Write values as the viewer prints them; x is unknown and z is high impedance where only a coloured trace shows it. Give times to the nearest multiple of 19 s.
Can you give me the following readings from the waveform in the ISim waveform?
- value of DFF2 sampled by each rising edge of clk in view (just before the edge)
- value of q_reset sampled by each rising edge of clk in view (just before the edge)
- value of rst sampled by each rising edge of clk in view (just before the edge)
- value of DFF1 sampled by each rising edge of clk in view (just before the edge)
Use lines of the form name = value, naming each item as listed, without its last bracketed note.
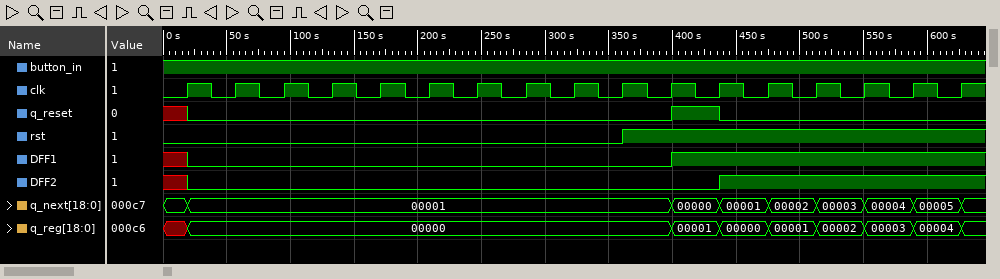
value of DFF2 sampled by each rising edge of clk in view = x 0 0 0 0 0 0 0 0 0 0 0 1 1 1 1 1
value of q_reset sampled by each rising edge of clk in view = x 0 0 0 0 0 0 0 0 0 0 1 0 0 0 0 0
value of rst sampled by each rising edge of clk in view = 0 0 0 0 0 0 0 0 0 0 1 1 1 1 1 1 1
value of DFF1 sampled by each rising edge of clk in view = x 0 0 0 0 0 0 0 0 0 0 1 1 1 1 1 1
